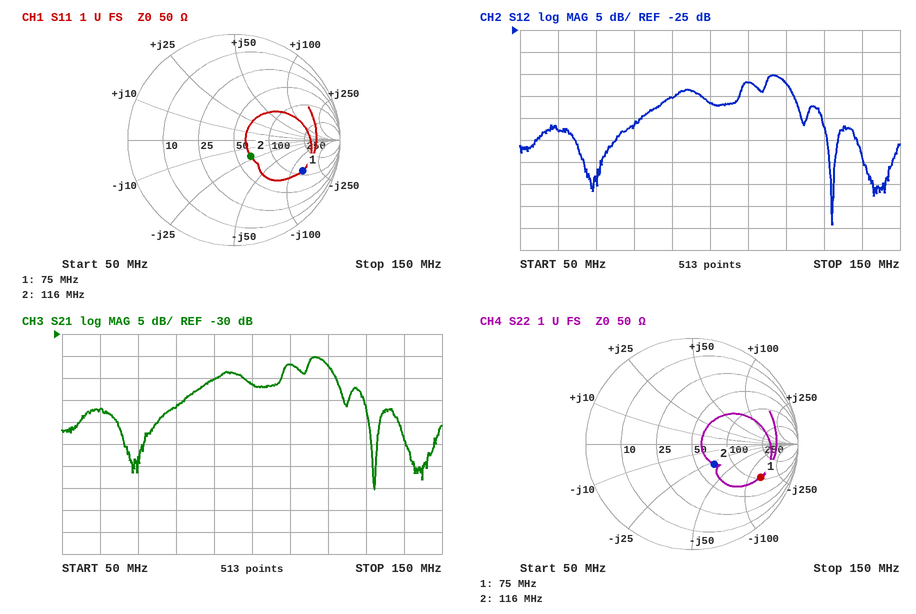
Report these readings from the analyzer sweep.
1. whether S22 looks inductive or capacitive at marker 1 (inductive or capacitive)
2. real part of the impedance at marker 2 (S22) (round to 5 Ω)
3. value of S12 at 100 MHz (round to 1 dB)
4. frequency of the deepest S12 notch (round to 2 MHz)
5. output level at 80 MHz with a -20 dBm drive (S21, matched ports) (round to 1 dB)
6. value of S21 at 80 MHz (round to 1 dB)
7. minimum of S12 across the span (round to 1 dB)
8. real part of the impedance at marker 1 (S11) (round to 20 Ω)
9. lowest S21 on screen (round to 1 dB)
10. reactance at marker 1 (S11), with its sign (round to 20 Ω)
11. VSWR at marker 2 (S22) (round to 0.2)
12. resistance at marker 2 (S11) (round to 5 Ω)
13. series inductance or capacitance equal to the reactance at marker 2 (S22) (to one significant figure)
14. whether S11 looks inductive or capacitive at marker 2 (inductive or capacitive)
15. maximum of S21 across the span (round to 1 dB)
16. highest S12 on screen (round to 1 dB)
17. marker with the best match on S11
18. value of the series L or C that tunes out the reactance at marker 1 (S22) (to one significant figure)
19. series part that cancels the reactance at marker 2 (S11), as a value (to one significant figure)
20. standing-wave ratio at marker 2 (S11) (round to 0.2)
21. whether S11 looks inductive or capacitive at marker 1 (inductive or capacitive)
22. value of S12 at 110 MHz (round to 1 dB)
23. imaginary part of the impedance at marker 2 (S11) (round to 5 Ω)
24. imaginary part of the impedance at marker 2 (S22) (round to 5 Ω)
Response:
capacitive
70 Ω
-42 dB
132 MHz
-67 dBm
-47 dB
-69 dB
120 Ω
-65 dB
-140 Ω
1.8
65 Ω
50 pF
capacitive
-35 dB
-35 dB
marker 2
300 nH
30 nH
1.6
capacitive
-37 dB
-20 Ω
-30 Ω
